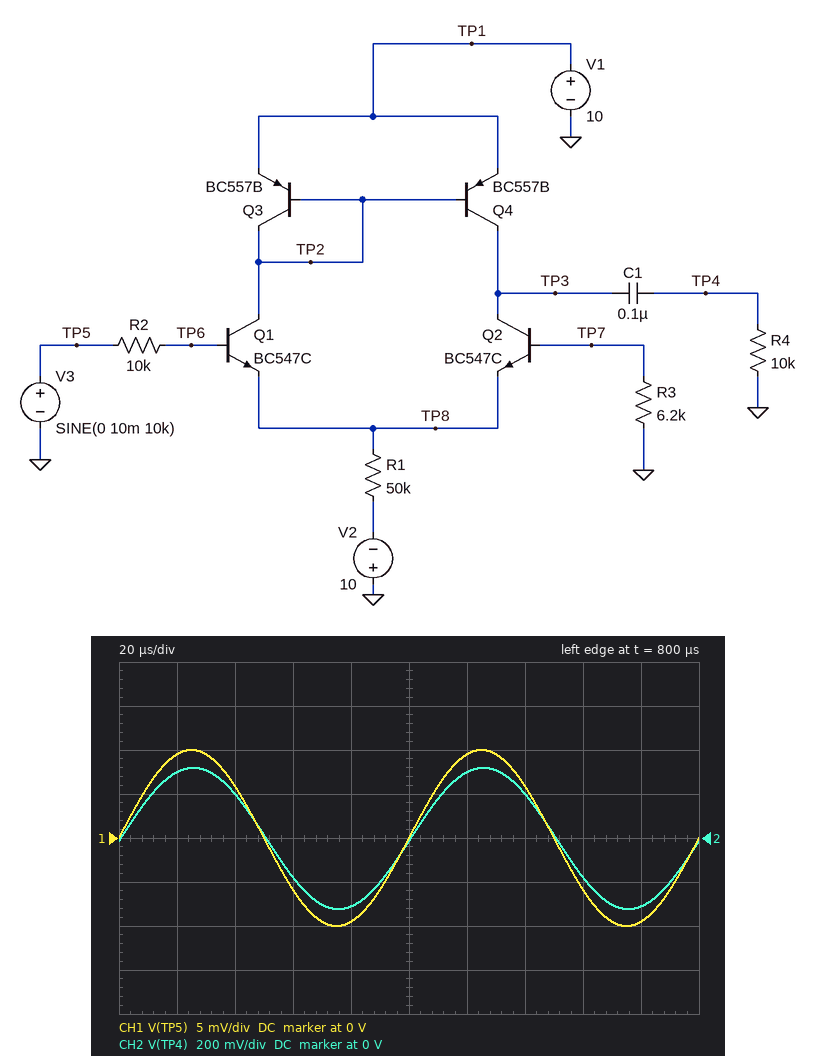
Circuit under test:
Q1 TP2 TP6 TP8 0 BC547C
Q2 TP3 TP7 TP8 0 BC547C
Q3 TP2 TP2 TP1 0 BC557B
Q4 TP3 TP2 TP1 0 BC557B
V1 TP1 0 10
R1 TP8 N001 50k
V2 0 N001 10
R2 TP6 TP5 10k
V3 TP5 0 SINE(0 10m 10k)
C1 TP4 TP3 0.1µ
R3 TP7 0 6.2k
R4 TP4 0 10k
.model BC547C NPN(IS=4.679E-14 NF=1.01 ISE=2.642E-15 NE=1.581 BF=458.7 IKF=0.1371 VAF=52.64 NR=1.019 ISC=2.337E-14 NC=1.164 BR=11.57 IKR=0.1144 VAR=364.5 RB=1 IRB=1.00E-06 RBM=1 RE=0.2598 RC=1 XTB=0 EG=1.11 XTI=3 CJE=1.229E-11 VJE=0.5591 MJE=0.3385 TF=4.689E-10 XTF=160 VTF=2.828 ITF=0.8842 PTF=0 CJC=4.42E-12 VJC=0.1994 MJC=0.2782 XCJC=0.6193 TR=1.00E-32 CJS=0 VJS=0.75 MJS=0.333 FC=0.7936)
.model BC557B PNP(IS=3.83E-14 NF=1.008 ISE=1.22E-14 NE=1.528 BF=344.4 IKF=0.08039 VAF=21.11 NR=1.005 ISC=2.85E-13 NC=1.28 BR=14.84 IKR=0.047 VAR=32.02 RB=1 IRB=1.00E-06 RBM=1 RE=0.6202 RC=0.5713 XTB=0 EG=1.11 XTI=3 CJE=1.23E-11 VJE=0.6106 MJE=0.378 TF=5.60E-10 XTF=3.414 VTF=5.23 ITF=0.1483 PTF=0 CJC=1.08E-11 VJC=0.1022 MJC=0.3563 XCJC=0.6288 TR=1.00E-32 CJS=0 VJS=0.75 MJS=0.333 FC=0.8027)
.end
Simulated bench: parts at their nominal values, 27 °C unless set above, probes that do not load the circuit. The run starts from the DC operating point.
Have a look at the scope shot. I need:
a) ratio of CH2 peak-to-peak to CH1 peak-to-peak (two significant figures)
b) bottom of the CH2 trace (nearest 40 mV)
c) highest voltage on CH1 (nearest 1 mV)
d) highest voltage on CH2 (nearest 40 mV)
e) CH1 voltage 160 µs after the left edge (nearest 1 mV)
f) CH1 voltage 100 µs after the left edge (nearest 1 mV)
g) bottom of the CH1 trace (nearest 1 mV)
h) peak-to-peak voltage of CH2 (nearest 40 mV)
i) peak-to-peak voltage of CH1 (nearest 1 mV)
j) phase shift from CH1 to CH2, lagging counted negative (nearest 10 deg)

32
-320 mV
10 mV
320 mV
-6 mV
0 V
-10 mV
640 mV
20 mV
0 deg
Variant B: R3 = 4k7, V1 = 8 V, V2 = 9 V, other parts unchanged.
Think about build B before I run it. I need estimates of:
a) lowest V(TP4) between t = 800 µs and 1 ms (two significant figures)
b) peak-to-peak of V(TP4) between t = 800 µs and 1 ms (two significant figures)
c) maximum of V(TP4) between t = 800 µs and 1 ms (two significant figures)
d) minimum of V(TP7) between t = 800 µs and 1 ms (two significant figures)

-290 mV
580 mV
290 mV
-1.0 mV
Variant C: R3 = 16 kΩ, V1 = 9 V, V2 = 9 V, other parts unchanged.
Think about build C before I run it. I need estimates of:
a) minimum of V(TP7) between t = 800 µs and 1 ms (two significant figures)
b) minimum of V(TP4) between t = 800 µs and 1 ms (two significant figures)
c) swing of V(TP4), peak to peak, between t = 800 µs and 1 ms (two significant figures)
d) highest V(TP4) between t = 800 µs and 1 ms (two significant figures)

-3.3 mV
-270 mV
420 mV
140 mV
